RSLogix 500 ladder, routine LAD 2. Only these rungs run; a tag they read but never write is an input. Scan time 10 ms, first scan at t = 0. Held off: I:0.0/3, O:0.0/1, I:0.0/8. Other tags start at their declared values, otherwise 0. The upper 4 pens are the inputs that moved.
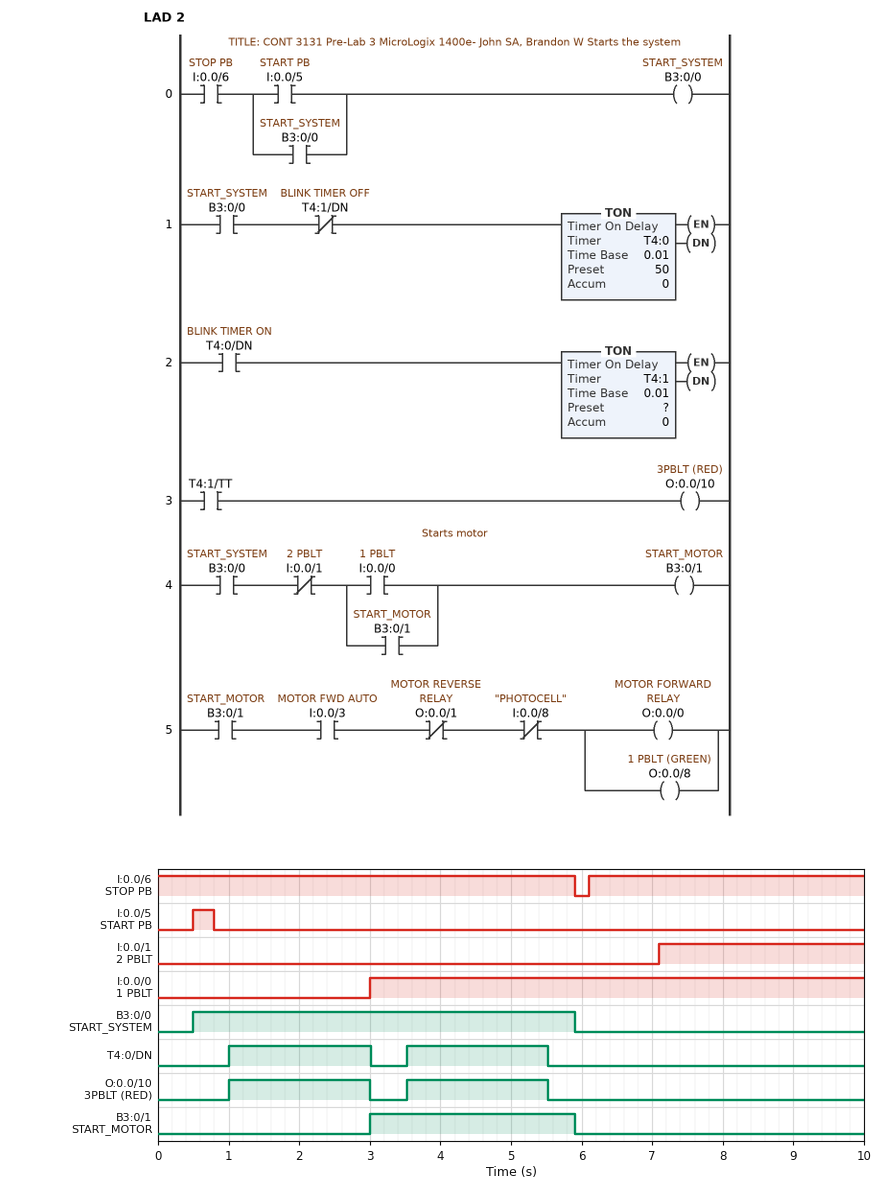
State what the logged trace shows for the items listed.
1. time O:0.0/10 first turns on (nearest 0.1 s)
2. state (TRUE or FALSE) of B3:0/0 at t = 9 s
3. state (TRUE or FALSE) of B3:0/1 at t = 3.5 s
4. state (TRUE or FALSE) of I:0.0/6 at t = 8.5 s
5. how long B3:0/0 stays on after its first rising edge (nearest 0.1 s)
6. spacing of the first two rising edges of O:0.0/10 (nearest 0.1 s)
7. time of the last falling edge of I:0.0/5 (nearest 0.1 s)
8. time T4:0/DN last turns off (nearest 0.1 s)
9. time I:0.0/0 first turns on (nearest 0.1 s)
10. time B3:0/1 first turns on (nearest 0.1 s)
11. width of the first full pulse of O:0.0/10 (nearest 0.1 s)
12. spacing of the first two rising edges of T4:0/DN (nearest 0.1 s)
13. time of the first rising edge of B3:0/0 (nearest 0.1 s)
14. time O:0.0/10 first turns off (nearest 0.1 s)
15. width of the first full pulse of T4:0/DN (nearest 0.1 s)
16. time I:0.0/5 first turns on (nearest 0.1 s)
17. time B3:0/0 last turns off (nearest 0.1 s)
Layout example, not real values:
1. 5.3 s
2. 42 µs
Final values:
1. 1.0 s
2. FALSE
3. TRUE
4. TRUE
5. 5.4 s
6. 2.5 s
7. 0.8 s
8. 5.5 s
9. 3.0 s
10. 3.0 s
11. 2.0 s
12. 2.5 s
13. 0.5 s
14. 3.0 s
15. 2.0 s
16. 0.5 s
17. 5.9 s
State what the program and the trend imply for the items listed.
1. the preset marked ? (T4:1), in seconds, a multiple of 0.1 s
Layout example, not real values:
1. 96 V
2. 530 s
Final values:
1. 2.0 s
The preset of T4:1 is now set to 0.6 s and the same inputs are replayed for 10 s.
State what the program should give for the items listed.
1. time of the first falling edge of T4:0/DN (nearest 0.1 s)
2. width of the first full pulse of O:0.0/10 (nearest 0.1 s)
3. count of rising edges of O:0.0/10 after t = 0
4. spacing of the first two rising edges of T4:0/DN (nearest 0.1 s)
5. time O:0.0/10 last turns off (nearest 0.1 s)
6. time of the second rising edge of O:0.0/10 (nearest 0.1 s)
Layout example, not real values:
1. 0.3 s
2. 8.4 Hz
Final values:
1. 1.6 s
2. 0.6 s
3. 5
4. 1.1 s
5. 5.9 s
6. 2.1 s
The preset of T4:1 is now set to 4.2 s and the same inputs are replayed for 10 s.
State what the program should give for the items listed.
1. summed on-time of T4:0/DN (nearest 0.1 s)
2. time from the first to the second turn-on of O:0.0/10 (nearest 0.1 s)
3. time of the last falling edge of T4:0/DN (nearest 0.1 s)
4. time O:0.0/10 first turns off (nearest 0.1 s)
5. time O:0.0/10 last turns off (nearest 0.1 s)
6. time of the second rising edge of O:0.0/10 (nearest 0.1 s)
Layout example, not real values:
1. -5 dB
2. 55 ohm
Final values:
1. 4.4 s
2. 4.7 s
3. 5.9 s
4. 5.2 s
5. 5.9 s
6. 5.7 s
